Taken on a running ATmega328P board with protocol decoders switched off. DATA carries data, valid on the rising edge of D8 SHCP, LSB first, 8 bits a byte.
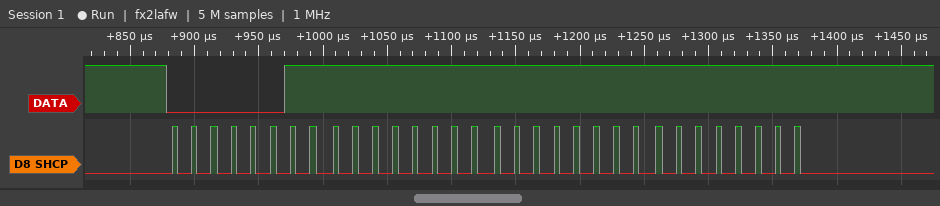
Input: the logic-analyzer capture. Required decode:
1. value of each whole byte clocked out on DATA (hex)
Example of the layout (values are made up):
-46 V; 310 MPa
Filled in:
C0 FF FF FF
